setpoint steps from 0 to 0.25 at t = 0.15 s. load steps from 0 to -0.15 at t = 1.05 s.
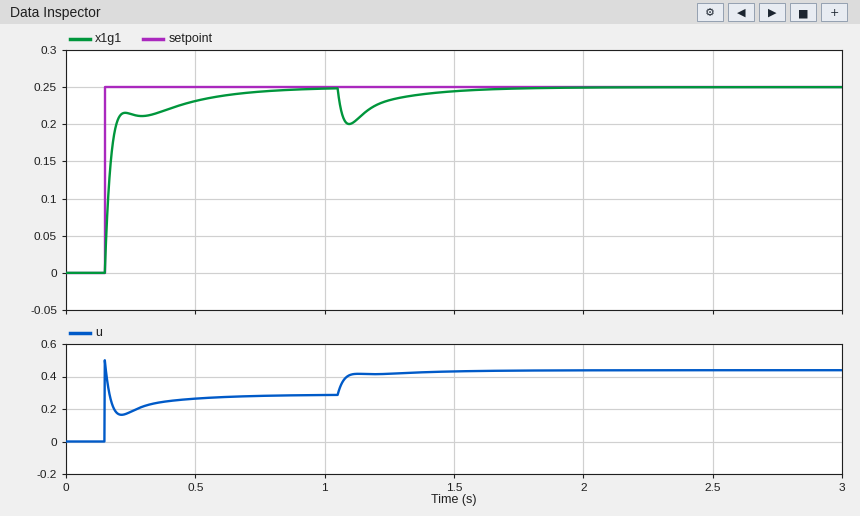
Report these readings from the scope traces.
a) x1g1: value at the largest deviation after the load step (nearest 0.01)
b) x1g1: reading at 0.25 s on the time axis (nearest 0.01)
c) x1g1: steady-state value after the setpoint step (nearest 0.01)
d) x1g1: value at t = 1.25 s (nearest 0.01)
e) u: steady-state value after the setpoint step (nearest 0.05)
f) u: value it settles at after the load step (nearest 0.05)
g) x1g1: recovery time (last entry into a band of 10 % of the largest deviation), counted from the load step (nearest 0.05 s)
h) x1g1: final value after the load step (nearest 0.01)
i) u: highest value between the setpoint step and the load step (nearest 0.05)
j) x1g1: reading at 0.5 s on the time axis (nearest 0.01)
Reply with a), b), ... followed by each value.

a) 0.20
b) 0.21
c) 0.25
d) 0.23
e) 0.30
f) 0.45
g) 0.50 s
h) 0.25
i) 0.50
j) 0.23
